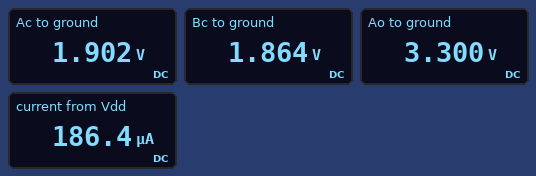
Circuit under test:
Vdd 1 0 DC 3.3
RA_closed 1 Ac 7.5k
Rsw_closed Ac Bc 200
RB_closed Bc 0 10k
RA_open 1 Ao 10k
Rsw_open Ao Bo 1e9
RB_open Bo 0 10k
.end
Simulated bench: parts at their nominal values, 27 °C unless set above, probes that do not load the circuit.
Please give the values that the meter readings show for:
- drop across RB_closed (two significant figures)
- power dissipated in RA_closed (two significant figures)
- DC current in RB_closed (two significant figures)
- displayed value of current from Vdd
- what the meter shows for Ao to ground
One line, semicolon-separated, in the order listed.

1.9 V; 260 µW; 190 µA; 186.4 µA; 3.300 V
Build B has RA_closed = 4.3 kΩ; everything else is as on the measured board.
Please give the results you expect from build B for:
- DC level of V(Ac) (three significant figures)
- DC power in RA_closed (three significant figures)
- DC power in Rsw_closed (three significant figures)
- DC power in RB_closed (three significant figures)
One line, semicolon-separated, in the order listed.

2.32 V; 223 µW; 10.4 µW; 518 µW
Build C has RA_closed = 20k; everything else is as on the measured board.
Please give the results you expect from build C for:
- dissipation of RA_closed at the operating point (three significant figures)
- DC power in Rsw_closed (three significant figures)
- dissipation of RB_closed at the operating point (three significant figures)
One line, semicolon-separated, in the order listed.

239 µW; 2.39 µW; 119 µW
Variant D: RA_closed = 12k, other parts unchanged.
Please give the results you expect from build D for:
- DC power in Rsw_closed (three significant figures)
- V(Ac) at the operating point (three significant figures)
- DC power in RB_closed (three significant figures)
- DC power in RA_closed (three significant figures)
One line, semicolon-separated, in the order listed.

4.42 µW; 1.52 V; 221 µW; 265 µW
